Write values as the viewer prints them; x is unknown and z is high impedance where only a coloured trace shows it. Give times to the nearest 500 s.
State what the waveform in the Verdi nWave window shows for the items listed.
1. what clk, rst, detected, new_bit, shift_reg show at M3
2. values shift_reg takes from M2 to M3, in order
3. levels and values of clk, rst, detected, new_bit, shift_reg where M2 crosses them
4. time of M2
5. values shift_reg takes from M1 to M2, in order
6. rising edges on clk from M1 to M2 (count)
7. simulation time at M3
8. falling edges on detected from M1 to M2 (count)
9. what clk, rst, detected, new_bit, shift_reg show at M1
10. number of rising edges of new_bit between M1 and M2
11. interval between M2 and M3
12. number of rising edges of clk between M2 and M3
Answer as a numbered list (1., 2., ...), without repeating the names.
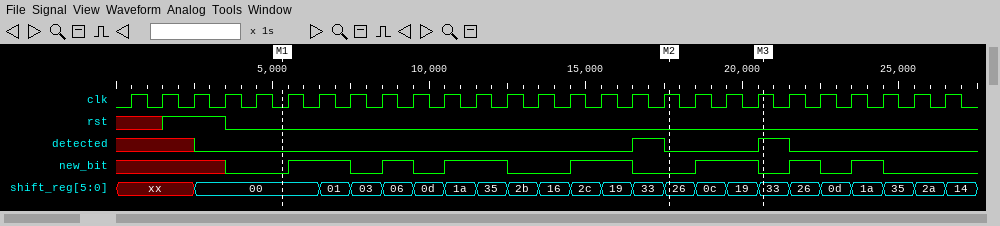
1. clk=1, rst=0, detected=1, new_bit=0, shift_reg=33
2. 26, 0c, 19, 33
3. clk=1, rst=0, detected=0, new_bit=0, shift_reg=26
4. 17500 s
5. 00, 01, 03, 06, 0d, 1a, 35, 2b, 16, 2c, 19, 33, 26
6. 13
7. 20500 s
8. 1
9. clk=0, rst=0, detected=0, new_bit=0, shift_reg=00
10. 4
11. 3000 s
12. 3
